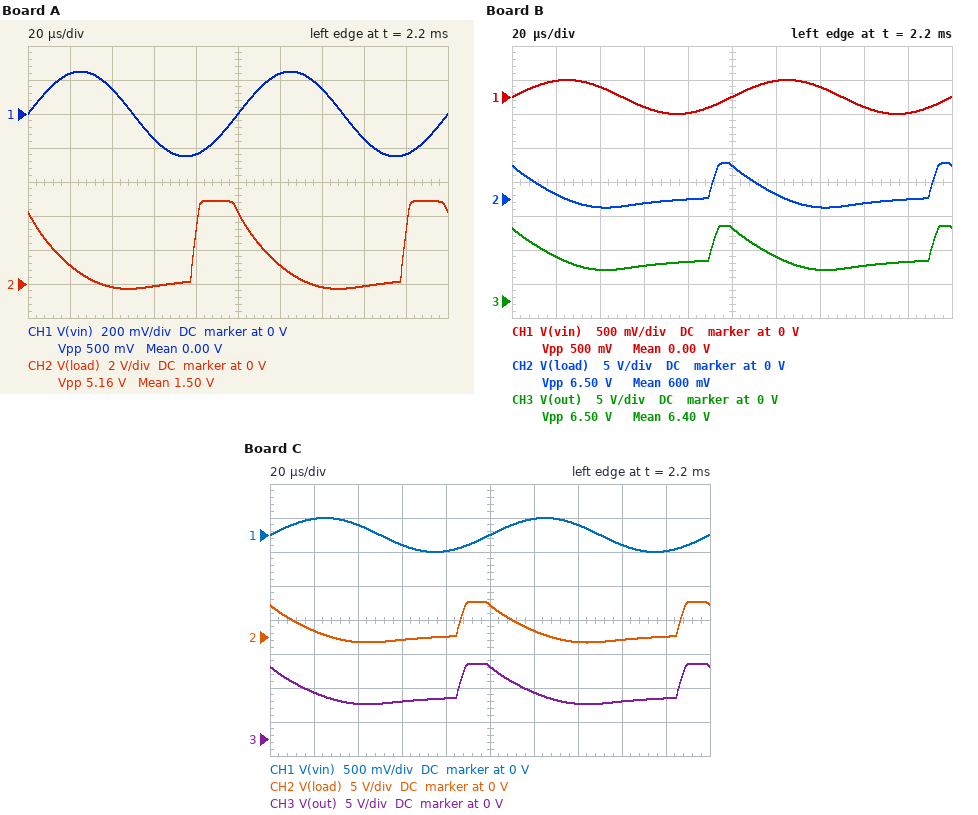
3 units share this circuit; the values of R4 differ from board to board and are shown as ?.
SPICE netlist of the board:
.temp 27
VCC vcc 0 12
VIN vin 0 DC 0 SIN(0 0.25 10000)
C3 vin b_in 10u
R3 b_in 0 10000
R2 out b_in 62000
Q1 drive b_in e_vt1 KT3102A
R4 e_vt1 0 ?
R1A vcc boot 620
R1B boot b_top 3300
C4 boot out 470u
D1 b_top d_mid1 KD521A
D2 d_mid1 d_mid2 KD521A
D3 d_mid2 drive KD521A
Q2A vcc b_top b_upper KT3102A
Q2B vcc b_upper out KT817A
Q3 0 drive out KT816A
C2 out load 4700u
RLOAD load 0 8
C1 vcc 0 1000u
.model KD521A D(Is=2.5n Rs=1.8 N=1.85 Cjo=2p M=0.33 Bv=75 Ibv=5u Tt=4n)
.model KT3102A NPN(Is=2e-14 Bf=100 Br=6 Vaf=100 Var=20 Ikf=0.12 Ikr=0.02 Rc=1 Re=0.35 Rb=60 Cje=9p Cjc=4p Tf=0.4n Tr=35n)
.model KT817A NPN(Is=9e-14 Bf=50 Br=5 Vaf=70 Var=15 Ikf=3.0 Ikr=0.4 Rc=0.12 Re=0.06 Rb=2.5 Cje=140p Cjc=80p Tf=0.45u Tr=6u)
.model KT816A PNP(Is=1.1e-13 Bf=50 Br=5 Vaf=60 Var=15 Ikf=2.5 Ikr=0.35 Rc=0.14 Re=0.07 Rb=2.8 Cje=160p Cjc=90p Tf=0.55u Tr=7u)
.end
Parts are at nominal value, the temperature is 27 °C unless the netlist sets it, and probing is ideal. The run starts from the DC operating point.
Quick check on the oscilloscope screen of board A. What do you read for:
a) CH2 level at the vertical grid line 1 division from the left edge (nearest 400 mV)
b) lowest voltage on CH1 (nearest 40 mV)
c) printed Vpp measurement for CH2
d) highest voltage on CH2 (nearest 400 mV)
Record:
1.2 V
-240 mV
5.16 V
4.8 V
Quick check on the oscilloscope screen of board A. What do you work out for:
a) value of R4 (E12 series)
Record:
68 Ω
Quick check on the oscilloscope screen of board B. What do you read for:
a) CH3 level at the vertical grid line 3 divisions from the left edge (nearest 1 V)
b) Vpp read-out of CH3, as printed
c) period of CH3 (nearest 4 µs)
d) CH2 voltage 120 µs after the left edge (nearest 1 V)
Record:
5 V
6.50 V
100 µs
1 V
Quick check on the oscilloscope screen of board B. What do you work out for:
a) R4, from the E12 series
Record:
22 Ω
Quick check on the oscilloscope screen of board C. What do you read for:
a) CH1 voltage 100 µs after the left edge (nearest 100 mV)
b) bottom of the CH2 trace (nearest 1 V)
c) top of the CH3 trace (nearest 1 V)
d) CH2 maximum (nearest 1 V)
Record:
0 V
-1 V
11 V
5 V
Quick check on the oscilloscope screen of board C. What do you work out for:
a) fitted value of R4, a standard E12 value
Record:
33 Ω
